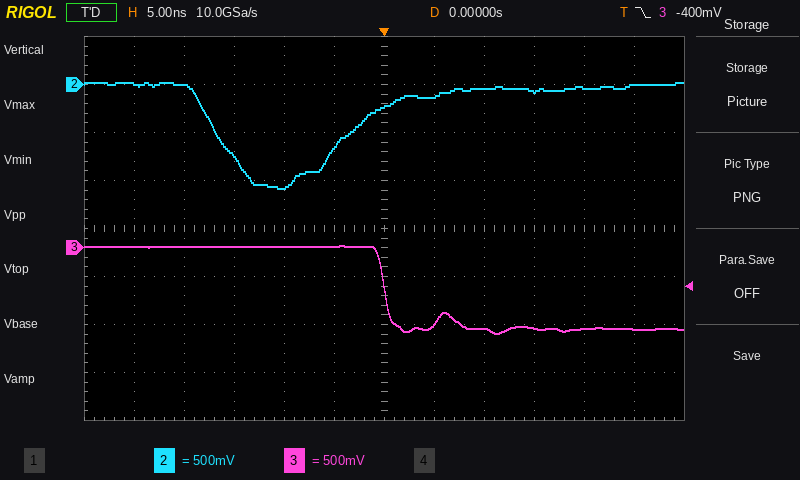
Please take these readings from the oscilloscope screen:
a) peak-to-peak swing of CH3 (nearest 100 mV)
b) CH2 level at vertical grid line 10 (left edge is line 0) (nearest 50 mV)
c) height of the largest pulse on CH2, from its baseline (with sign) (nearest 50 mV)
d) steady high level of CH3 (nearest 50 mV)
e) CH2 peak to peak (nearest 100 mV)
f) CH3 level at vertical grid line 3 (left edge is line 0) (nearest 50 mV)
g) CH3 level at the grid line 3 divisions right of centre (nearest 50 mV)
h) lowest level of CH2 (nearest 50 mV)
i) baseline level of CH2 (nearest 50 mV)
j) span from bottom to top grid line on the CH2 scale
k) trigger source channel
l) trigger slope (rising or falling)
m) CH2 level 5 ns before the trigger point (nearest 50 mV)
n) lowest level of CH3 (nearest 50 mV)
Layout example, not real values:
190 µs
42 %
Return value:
900 mV
-50 mV
-1.05 V
0 mV
1.10 V
0 mV
-850 mV
-1.10 V
-50 mV
4 V
CH3
falling
-650 mV
-900 mV
